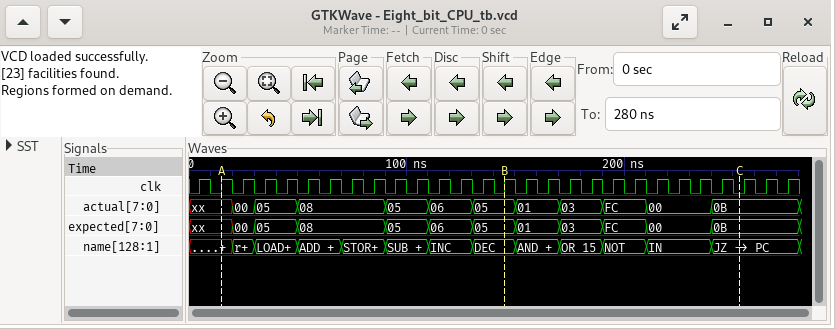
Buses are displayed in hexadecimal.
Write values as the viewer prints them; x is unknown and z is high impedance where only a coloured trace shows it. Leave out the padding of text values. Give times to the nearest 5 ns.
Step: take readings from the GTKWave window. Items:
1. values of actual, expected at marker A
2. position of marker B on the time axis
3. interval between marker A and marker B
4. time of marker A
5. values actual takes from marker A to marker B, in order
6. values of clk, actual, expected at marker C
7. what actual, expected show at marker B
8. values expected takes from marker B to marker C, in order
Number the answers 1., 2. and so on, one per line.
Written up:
1. actual=xx, expected=xx
2. 145 ns
3. 130 ns
4. 15 ns
5. xx, 00, 05, 08, 05, 06, 05
6. clk=0, actual=0B, expected=0B
7. actual=05, expected=05
8. 05, 01, 03, FC, 00, 0B
